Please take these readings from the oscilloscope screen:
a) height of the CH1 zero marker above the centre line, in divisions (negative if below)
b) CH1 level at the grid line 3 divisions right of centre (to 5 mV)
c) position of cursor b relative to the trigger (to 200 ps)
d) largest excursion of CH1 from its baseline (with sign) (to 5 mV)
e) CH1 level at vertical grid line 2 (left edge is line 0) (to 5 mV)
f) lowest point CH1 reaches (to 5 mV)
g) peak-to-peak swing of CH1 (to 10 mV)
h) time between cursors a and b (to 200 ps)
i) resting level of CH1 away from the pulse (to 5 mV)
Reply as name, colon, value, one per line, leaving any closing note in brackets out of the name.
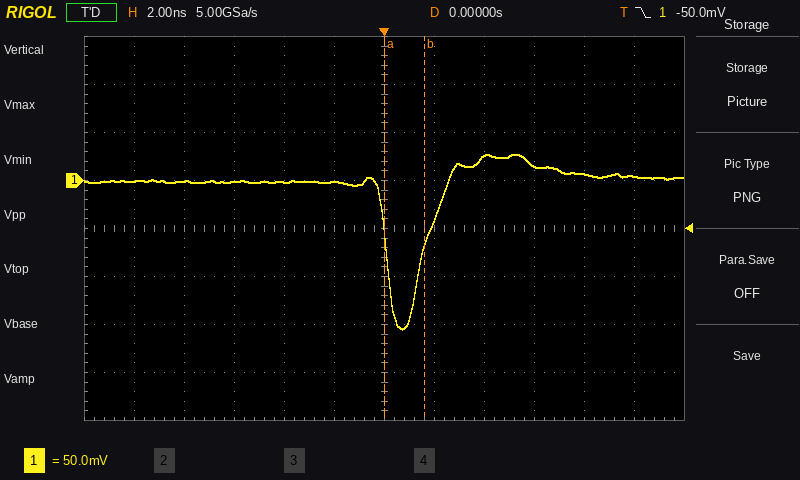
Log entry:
height of the CH1 zero marker above the centre line, in divisions: +1.0 div
CH1 level at the grid line 3 divisions right of centre: 15 mV
position of cursor b relative to the trigger: +1.6 ns
largest excursion of CH1 from its baseline (with sign): -155 mV
CH1 level at vertical grid line 2 (left edge is line 0): 0 mV
lowest point CH1 reaches: -155 mV
peak-to-peak swing of CH1: 180 mV
time between cursors a and b: 1.6 ns
resting level of CH1 away from the pulse: 0 mV
